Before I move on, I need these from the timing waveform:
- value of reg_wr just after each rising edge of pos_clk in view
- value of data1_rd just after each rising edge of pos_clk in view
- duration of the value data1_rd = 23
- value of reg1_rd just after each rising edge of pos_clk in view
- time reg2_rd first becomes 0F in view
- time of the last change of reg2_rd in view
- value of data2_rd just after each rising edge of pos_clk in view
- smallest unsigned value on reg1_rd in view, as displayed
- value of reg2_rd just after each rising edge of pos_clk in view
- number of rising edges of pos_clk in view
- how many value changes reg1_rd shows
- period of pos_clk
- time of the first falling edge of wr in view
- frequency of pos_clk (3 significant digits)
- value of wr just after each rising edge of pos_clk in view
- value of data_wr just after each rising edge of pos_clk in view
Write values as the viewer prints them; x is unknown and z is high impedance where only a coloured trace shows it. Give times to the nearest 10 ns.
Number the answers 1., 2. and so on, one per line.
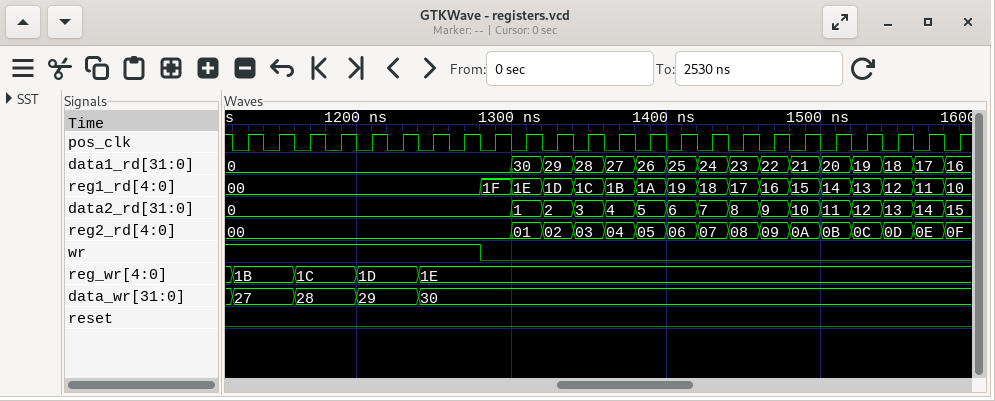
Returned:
1. 1B, 1B, 1C, 1C, 1D, 1D, 1E, 1E, 1E, 1E, 1E, 1E, 1E, 1E, 1E, 1E, 1E, 1E, 1E, 1E, 1E, 1E, 1E, 1E
2. 0, 0, 0, 0, 0, 0, 0, 0, 0, 30, 29, 28, 27, 26, 25, 24, 23, 22, 21, 20, 19, 18, 17, 16
3. 20 ns
4. 00, 00, 00, 00, 00, 00, 00, 00, 1F, 1E, 1D, 1C, 1B, 1A, 19, 18, 17, 16, 15, 14, 13, 12, 11, 10
5. 1580 ns
6. 1580 ns
7. 0, 0, 0, 0, 0, 0, 0, 0, 0, 1, 2, 3, 4, 5, 6, 7, 8, 9, 10, 11, 12, 13, 14, 15
8. 00
9. 00, 00, 00, 00, 00, 00, 00, 00, 00, 01, 02, 03, 04, 05, 06, 07, 08, 09, 0A, 0B, 0C, 0D, 0E, 0F
10. 24
11. 16
12. 20 ns
13. 1280 ns
14. 50.0 MHz
15. 1 1 1 1 1 1 1 1 0 0 0 0 0 0 0 0 0 0 0 0 0 0 0 0
16. 27, 27, 28, 28, 29, 29, 30, 30, 30, 30, 30, 30, 30, 30, 30, 30, 30, 30, 30, 30, 30, 30, 30, 30
